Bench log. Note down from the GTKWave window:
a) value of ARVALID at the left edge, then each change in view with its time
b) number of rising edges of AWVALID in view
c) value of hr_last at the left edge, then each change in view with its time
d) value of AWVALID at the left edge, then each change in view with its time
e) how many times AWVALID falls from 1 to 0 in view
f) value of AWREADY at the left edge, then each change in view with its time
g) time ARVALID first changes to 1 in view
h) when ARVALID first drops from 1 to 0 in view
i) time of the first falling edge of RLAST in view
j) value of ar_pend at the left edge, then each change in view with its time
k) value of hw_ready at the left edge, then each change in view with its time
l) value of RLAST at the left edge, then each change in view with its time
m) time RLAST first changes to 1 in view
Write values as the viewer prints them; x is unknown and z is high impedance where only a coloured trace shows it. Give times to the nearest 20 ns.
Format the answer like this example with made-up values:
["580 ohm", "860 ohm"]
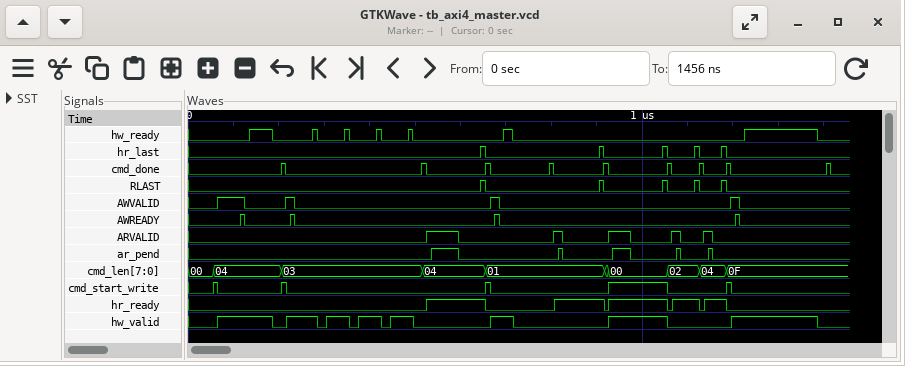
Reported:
["0, 1 at 520 ns, 0 at 600 ns, 1 at 800 ns, 0 at 820 ns, 1 at 920 ns, 0 at 980 ns, 1 at 1060 ns, 0 at 1080 ns, 1 at 1140 ns, 0 at 1160 ns", "4", "0, 1 at 640 ns, 0 at 660 ns, 1 at 900 ns, 0 at 920 ns, 1 at 1040 ns, 0 at 1060 ns, 1 at 1120 ns, 0 at 1120 ns, 1 at 1180 ns, 0 at 1180 ns", "0, 1 at 60 ns, 0 at 120 ns, 1 at 220 ns, 0 at 240 ns, 1 at 660 ns, 0 at 680 ns, 1 at 1200 ns, 0 at 1220 ns", "4", "0, 1 at 120 ns, 0 at 120 ns, 1 at 220 ns, 0 at 240 ns, 1 at 680 ns, 0 at 680 ns, 1 at 1200 ns, 0 at 1220 ns", "520 ns", "600 ns", "660 ns", "0, 1 at 540 ns, 0 at 600 ns, 1 at 820 ns, 0 at 820 ns, 1 at 940 ns, 0 at 980 ns, 1 at 1080 ns, 0 at 1080 ns, 1 at 1140 ns, 0 at 1160 ns", "0, 1 at 140 ns, 0 at 180 ns, 1 at 280 ns, 0 at 280 ns, 1 at 340 ns, 0 at 360 ns, 1 at 420 ns, 0 at 420 ns, 1 at 480 ns, 0 at 500 ns, 1 at 700 ns, 0 at 720 ns, 1 at 1220 ns, 0 at 1380 ns", "0, 1 at 640 ns, 0 at 660 ns, 1 at 900 ns, 0 at 920 ns, 1 at 1040 ns, 0 at 1060 ns, 1 at 1120 ns, 0 at 1120 ns, 1 at 1180 ns, 0 at 1180 ns", "640 ns"]
